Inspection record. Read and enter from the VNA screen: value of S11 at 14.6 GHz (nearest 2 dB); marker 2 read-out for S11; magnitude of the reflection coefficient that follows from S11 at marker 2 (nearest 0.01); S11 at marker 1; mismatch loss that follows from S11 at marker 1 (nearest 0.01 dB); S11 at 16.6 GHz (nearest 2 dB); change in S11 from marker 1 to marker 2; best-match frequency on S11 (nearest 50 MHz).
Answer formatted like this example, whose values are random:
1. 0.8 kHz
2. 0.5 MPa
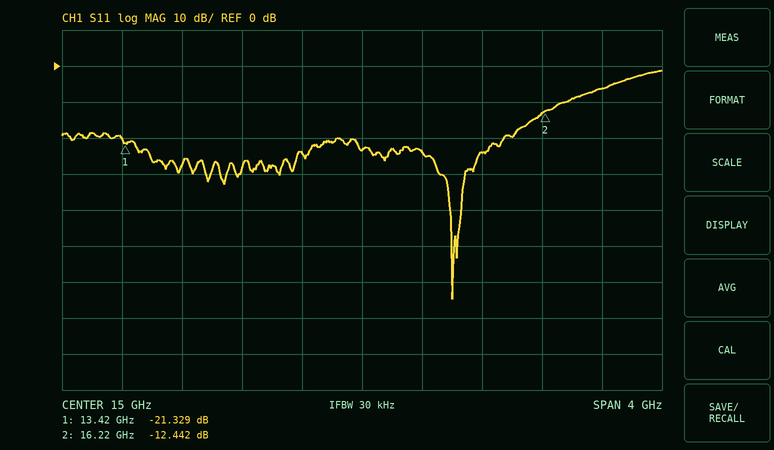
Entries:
1. -24 dB
2. -12.442 dB
3. 0.24
4. -21.329 dB
5. 0.03 dB
6. -6 dB
7. 8.887 dB
8. 15.60 GHz
